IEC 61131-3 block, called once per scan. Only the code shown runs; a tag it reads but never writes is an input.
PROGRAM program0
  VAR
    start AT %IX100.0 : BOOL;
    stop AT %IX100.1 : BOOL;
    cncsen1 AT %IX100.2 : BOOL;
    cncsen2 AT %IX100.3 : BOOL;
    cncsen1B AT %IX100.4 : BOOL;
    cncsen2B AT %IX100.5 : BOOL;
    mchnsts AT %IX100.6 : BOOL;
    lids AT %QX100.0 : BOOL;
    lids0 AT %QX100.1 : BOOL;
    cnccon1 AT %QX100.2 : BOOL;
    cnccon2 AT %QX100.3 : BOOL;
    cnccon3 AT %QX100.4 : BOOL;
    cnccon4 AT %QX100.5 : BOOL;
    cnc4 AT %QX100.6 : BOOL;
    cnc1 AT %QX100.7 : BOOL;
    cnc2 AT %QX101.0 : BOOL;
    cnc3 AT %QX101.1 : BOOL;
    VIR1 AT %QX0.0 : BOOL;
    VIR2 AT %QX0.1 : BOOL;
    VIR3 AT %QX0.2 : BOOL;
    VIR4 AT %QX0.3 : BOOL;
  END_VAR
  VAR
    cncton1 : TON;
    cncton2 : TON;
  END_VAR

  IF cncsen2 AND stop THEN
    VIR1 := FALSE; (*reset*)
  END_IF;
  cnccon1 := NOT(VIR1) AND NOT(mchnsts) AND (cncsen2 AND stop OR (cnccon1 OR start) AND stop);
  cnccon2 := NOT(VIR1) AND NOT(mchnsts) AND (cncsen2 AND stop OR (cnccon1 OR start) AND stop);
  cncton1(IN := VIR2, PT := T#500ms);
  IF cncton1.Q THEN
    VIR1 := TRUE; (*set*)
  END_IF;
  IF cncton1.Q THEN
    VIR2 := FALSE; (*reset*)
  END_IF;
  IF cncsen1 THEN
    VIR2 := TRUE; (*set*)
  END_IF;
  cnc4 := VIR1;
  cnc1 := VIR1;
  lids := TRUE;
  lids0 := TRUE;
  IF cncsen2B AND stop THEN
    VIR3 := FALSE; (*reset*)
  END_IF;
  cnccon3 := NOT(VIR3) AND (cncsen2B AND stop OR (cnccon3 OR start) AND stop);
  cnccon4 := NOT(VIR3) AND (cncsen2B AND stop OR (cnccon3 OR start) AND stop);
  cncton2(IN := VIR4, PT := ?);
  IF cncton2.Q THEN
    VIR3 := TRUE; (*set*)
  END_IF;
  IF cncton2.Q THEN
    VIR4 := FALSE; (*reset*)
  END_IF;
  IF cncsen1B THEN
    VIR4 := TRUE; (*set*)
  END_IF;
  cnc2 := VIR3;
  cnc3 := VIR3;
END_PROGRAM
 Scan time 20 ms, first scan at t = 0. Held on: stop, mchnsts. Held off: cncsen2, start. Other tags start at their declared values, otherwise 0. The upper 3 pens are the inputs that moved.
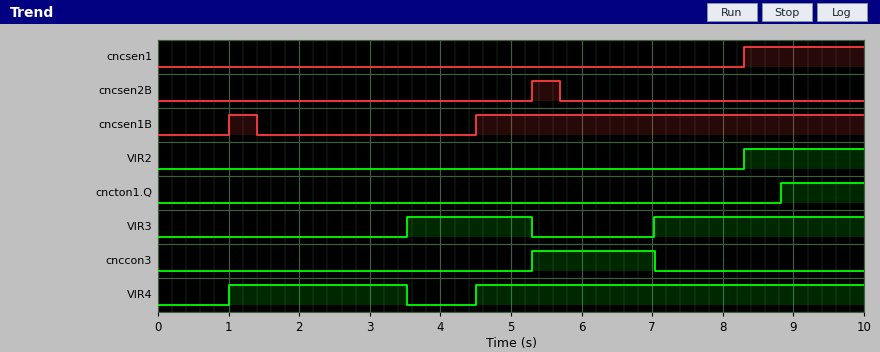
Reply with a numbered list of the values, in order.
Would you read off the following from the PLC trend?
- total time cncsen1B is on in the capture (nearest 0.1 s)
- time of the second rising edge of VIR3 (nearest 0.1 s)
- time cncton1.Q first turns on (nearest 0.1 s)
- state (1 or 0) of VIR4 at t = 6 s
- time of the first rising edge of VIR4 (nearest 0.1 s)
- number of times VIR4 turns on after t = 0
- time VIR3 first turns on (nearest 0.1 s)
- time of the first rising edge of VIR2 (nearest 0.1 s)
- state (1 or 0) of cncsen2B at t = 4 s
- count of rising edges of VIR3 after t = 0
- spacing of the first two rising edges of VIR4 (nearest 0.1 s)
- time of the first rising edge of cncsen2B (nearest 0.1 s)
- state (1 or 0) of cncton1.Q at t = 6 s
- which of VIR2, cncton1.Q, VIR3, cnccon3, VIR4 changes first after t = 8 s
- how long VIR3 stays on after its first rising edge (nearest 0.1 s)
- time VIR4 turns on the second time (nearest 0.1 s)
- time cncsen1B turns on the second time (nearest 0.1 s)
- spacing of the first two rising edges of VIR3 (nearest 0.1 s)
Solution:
1. 5.9 s
2. 7.0 s
3. 8.8 s
4. 1
5. 1.0 s
6. 2
7. 3.5 s
8. 8.3 s
9. 0
10. 2
11. 3.5 s
12. 5.3 s
13. 0
14. VIR2
15. 1.8 s
16. 4.5 s
17. 4.5 s
18. 3.5 s
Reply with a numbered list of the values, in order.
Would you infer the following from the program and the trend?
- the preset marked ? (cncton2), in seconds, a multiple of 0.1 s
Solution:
1. 2.5 s
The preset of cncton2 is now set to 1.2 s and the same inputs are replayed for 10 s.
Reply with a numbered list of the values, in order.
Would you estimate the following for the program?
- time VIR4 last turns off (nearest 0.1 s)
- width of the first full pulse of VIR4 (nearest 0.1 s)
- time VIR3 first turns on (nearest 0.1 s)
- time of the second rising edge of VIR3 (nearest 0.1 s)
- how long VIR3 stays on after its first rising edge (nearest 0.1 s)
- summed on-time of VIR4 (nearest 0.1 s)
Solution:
1. 2.2 s
2. 1.2 s
3. 2.2 s
4. 5.7 s
5. 3.1 s
6. 6.7 s
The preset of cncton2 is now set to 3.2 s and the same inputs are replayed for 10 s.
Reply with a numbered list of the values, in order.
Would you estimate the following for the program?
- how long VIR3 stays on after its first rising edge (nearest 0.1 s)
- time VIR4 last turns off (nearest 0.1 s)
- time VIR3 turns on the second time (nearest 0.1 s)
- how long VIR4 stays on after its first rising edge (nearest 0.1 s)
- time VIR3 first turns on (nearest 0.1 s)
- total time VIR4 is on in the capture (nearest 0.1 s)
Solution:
1. 1.1 s
2. 4.2 s
3. 7.7 s
4. 3.2 s
5. 4.2 s
6. 8.7 s
